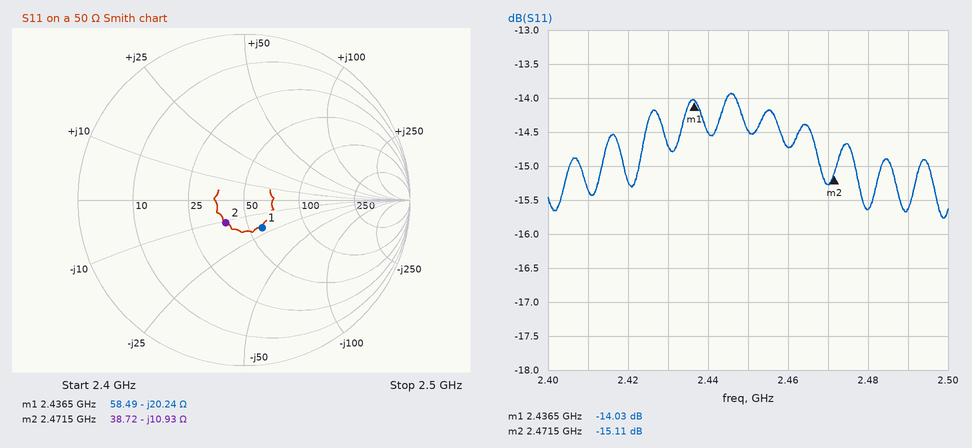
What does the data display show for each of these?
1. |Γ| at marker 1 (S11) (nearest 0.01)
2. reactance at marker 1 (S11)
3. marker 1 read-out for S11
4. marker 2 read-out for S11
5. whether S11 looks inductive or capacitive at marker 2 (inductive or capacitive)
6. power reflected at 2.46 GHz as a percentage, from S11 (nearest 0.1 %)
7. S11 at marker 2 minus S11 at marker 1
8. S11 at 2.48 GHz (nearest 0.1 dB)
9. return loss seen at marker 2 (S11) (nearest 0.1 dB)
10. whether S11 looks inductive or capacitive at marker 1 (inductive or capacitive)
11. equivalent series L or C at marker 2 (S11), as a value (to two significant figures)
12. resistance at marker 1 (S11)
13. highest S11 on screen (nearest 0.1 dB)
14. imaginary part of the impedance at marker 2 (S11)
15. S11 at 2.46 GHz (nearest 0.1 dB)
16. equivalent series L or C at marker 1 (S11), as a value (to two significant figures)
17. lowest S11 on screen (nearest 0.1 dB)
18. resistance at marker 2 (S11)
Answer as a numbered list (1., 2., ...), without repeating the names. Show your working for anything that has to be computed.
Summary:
1. 0.20
2. -20.24 Ω
3. -14.03 dB
4. -15.11 dB
5. capacitive
6. 10^(-14.7/10) ≈ 3.4 %
7. -15.11 − (-14.03) = -1.08 dB
8. -15.6 dB
9. 15.1 dB
10. capacitive
11. C = 1/(2π × 2.4715 GHz × 10.93 Ω) ≈ 5.9 pF
12. 58.49 Ω
13. -13.9 dB
14. -10.93 Ω
15. -14.7 dB
16. C = 1/(2π × 2.4365 GHz × 20.24 Ω) ≈ 3.2 pF
17. -15.8 dB
18. 38.72 Ω
